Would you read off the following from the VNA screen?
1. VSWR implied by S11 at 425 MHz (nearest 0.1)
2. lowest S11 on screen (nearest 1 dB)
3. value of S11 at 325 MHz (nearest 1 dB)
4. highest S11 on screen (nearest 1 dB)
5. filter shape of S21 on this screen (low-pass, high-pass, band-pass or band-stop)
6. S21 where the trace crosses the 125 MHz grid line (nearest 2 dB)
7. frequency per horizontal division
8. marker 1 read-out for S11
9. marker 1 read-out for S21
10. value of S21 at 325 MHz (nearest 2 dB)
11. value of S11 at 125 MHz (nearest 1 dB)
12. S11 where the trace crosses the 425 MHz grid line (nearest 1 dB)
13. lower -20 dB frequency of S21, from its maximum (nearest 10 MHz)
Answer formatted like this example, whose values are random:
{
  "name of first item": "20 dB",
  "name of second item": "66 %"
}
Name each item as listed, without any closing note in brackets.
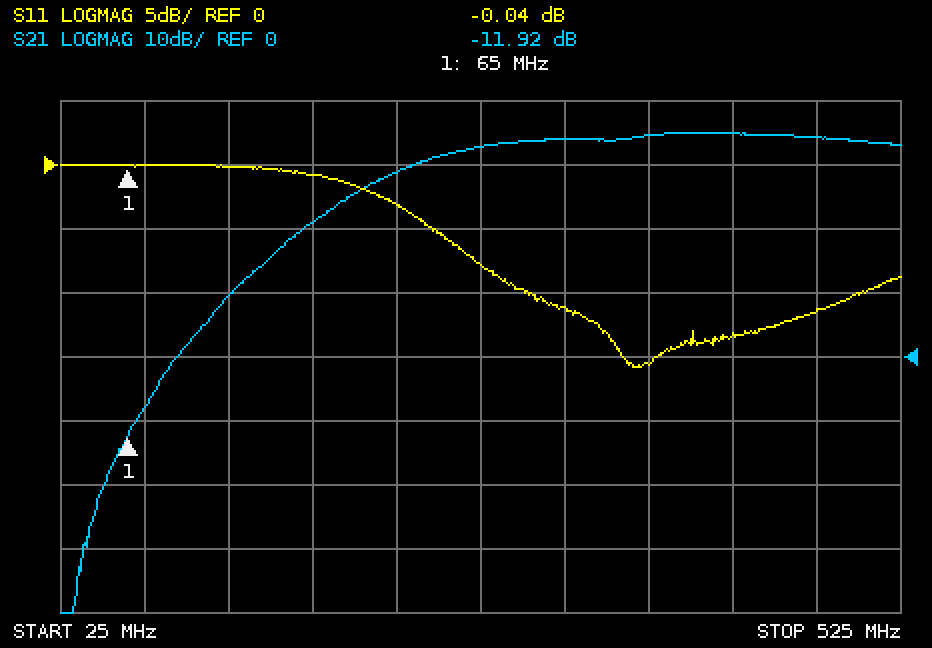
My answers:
{
  "VSWR implied by S11 at 425 MHz": "1.6",
  "lowest S11 on screen": "-16 dB",
  "value of S11 at 325 MHz": "-11 dB",
  "highest S11 on screen": "0 dB",
  "filter shape of S21 on this screen": "high-pass",
  "S21 where the trace crosses the 125 MHz grid line": "10 dB",
  "frequency per horizontal division": "50 MHz",
  "marker 1 read-out for S11": "-0.04 dB",
  "marker 1 read-out for S21": "-11.92 dB",
  "value of S21 at 325 MHz": "34 dB",
  "value of S11 at 125 MHz": "0 dB",
  "S11 where the trace crosses the 425 MHz grid line": "-13 dB",
  "lower -20 dB frequency of S21, from its maximum": "150 MHz"
}
